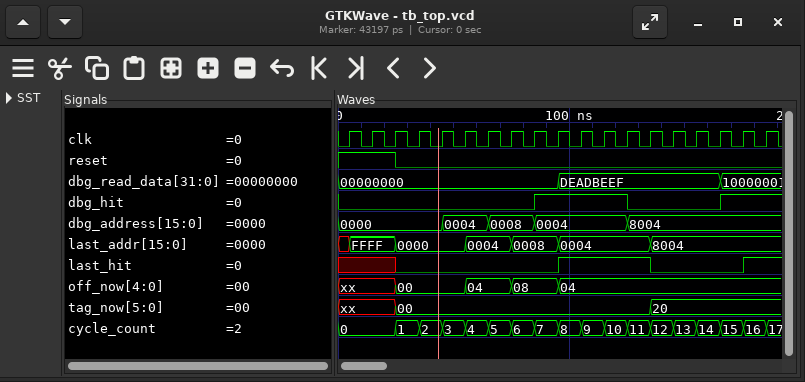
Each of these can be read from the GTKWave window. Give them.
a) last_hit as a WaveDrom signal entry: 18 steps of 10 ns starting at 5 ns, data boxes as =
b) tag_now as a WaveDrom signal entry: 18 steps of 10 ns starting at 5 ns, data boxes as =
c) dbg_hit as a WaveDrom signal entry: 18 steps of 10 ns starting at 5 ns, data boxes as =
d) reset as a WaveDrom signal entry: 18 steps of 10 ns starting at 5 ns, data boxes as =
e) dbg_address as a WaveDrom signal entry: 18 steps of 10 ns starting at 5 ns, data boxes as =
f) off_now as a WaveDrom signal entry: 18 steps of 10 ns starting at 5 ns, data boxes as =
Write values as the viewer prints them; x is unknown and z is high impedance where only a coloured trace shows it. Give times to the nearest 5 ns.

{name: 'last_hit', wave: 'x.0......1...0...1'}
{name: 'tag_now', wave: 'x.=..........=....', data: '00 20'}
{name: 'dbg_hit', wave: '0.......1...0...1.'}
{name: 'reset', wave: '1.0...............'}
{name: 'dbg_address', wave: '=...=.=.=...=.....', data: '0000 0004 0008 0004 8004'}
{name: 'off_now', wave: 'x.=..=.=.=........', data: '00 04 08 04'}
